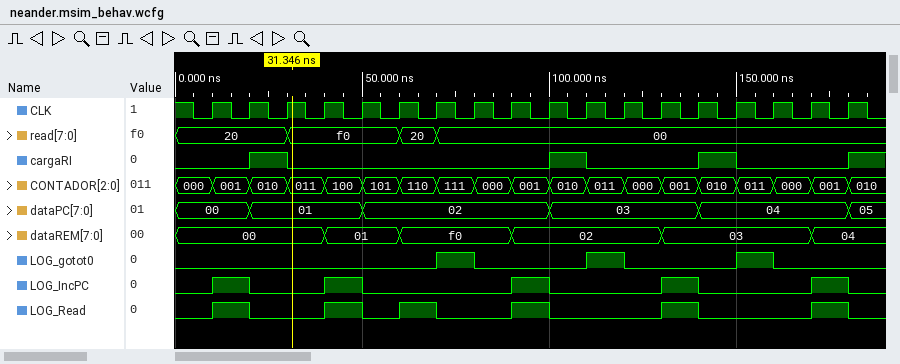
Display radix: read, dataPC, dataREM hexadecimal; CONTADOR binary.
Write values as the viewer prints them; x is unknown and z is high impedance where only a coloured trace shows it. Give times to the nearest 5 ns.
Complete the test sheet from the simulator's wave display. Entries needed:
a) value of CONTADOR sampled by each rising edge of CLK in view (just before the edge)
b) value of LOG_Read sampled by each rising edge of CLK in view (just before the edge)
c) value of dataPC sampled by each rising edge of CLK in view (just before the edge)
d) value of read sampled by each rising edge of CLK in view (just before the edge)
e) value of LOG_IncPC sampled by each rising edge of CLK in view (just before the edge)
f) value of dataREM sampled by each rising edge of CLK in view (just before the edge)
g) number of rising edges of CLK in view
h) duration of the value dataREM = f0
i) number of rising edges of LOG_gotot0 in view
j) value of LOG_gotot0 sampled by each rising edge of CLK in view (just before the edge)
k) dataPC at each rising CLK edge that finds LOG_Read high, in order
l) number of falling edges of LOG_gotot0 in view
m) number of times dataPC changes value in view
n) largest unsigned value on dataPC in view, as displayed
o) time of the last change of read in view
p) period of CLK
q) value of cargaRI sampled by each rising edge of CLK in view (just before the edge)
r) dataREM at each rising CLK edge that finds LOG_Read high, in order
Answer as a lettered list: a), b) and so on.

a) 000, 001, 010, 011, 100, 101, 110, 111, 000, 001, 010, 011, 000, 001, 010, 011, 000, 001
b) 0 1 0 0 1 0 1 0 0 1 0 0 0 1 0 0 0 1
c) 00, 00, 01, 01, 01, 02, 02, 02, 02, 02, 03, 03, 03, 03, 04, 04, 04, 04
d) 20, 20, 20, f0, f0, f0, 20, 00, 00, 00, 00, 00, 00, 00, 00, 00, 00, 00
e) 0 1 0 0 1 0 0 0 0 1 0 0 0 1 0 0 0 1
f) 00, 00, 00, 00, 01, 01, f0, f0, f0, 02, 02, 02, 02, 03, 03, 03, 03, 04
g) 18
h) 30 ns
i) 3
j) 0 0 0 0 0 0 0 1 0 0 0 1 0 0 0 1 0 0
k) 00, 01, 02, 02, 03, 04
l) 3
m) 5
n) 05
o) 70 ns
p) 10 ns
q) 0 0 1 0 0 0 0 0 0 0 1 0 0 0 1 0 0 0
r) 00, 01, f0, 02, 03, 04
